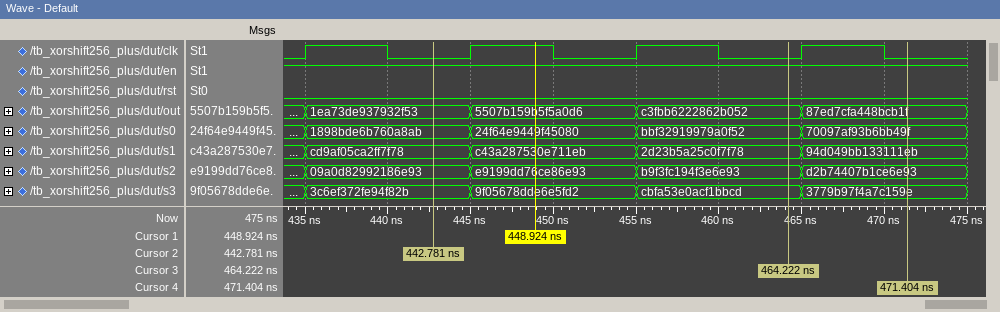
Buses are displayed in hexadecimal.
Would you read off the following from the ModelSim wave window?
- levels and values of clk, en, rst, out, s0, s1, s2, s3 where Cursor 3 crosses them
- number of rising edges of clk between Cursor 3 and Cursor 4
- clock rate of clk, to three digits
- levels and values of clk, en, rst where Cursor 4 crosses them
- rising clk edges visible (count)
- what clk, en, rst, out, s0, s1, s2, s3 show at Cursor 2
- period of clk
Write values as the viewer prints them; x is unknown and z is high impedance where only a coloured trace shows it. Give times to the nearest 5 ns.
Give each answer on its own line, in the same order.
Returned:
clk=0, en=1, rst=0, out=c3fbb6222862b052, s0=bbf32919979a0f52, s1=2d23b5a25c0f7f78, s2=b9f3fc194f3e6e93, s3=cbfa53e0acf1bbcd
1
100 MHz
clk=0, en=1, rst=0
4
clk=0, en=1, rst=0, out=1ea73de937932f53, s0=1898bde6b760a8ab, s1=cd9af05ca2ff7f78, s2=09a0d82992186e93, s3=3c6ef372fe94f82b
10 ns
